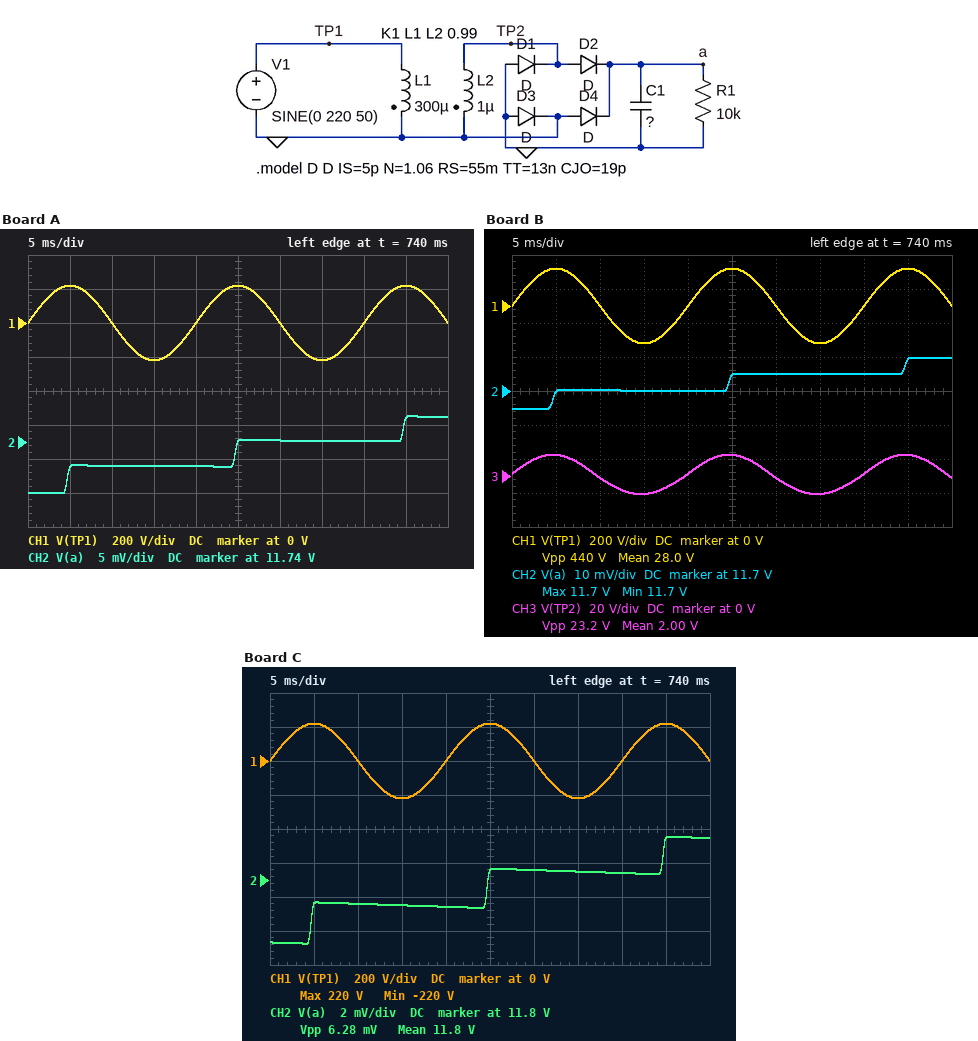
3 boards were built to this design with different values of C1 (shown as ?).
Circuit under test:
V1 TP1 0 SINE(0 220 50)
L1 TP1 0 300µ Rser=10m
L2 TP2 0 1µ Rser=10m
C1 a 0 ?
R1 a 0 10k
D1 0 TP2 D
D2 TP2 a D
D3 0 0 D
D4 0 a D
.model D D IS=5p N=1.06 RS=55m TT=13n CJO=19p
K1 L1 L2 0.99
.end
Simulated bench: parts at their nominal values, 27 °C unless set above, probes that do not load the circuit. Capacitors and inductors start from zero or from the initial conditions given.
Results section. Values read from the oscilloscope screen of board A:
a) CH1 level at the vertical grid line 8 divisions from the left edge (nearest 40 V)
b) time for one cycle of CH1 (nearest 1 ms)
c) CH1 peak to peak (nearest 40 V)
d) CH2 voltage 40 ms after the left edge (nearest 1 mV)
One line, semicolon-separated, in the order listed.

0 V; 20 ms; 440 V; 11.740 V
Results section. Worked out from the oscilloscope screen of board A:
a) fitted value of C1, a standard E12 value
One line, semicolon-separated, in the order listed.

120 mF
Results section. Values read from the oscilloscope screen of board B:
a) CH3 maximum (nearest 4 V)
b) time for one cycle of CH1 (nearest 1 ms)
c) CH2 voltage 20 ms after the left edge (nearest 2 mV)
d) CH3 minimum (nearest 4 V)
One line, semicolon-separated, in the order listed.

12 V; 20 ms; 11.700 V; -12 V
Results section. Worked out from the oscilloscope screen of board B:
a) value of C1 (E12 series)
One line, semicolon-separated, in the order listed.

150 mF
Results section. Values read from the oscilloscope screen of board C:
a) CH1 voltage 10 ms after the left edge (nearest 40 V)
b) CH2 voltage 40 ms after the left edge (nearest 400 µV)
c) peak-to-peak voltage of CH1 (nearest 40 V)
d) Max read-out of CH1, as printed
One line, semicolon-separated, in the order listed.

0 V; 11.7964 V; 440 V; 220 V
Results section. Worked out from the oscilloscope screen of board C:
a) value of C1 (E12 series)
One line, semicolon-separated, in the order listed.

68 mF
